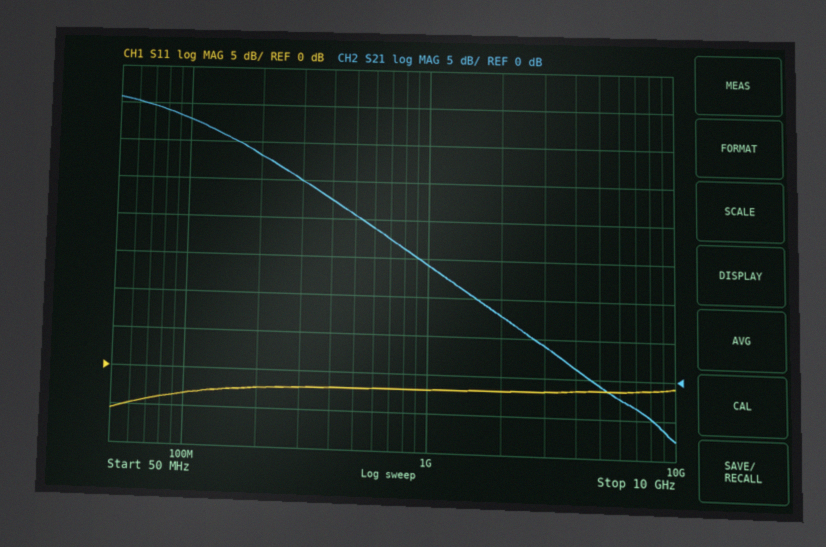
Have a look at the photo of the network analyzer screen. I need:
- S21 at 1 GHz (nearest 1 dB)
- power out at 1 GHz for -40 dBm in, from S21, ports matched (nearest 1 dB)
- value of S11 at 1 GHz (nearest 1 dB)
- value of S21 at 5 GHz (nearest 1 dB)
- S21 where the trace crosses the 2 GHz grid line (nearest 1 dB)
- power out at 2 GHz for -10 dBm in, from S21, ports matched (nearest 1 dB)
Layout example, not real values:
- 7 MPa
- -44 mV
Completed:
- 14 dB
- -26 dBm
- -2 dB
- -1 dB
- 8 dB
- -2 dBm
